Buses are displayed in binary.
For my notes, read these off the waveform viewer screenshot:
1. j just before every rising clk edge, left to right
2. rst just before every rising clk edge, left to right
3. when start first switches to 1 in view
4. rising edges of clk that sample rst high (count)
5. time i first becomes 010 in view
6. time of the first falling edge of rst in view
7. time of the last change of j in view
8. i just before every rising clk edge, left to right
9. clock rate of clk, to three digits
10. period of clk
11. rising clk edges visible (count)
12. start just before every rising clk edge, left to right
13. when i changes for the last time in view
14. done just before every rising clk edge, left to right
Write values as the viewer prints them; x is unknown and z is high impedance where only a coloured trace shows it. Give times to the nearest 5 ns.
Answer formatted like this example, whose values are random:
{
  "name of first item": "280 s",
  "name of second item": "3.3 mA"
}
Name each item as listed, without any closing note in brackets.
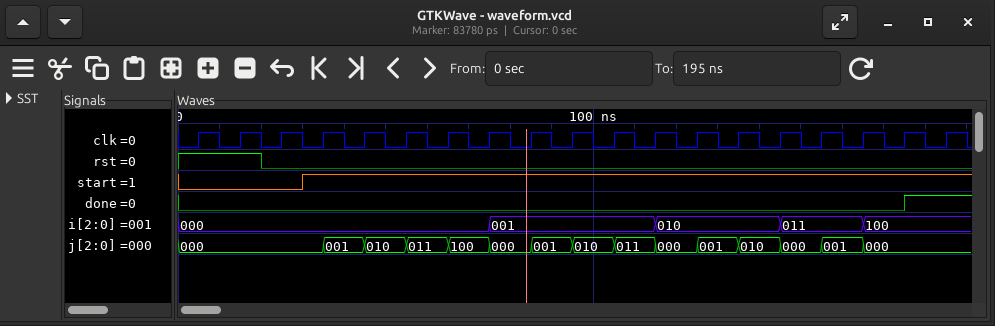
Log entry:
{
  "j just before every rising clk edge, left to right": "000, 000, 000, 000, 001, 010, 011, 100, 000, 001, 010, 011, 000, 001, 010, 000, 001, 000, 000",
  "rst just before every rising clk edge, left to right": "1 1 0 0 0 0 0 0 0 0 0 0 0 0 0 0 0 0 0",
  "when start first switches to 1 in view": "30 ns",
  "rising edges of clk that sample rst high": "2",
  "time i first becomes 010 in view": "115 ns",
  "time of the first falling edge of rst in view": "20 ns",
  "time of the last change of j in view": "165 ns",
  "i just before every rising clk edge, left to right": "000, 000, 000, 000, 000, 000, 000, 000, 001, 001, 001, 001, 010, 010, 010, 011, 011, 100, 100",
  "clock rate of clk, to three digits": "100 MHz",
  "period of clk": "10 ns",
  "rising clk edges visible": "19",
  "start just before every rising clk edge, left to right": "0 0 0 1 1 1 1 1 1 1 1 1 1 1 1 1 1 1 1",
  "when i changes for the last time in view": "165 ns",
  "done just before every rising clk edge, left to right": "0 0 0 0 0 0 0 0 0 0 0 0 0 0 0 0 0 0 1"
}
